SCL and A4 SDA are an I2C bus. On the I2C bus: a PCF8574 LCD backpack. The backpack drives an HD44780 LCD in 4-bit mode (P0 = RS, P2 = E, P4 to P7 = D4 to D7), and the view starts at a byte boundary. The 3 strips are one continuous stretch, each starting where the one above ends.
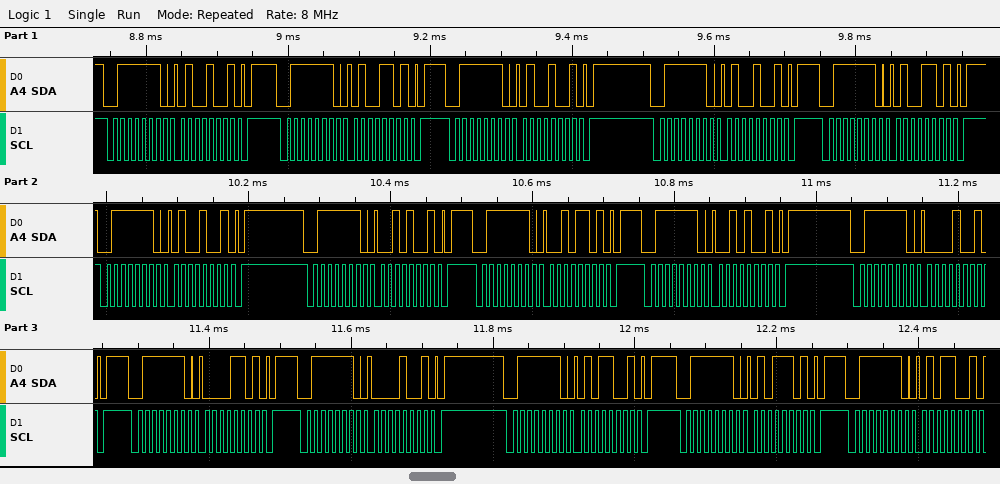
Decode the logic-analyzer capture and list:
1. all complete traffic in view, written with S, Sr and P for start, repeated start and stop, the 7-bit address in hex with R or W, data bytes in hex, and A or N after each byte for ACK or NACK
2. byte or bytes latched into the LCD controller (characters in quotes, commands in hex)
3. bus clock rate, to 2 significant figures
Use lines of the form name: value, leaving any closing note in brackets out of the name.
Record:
all complete traffic in view, written with S, Sr and P for start, repeated start and stop, the 7-bit address in hex with R or W, data bytes in hex, and A or N after each byte for ACK or NACK: S 3FW A 49 A P S 3FW A 4D A P S 3FW A 49 A P S 3FW A 49 A P S 3FW A 4D A P S 3FW A 49 A P S 3FW A 29 A P S 3FW A 2D A P S 3FW A 29 A P S 3FW A 09 A P S 3FW A 0D A P S 3FW A 09 A P S 3FW A 59 A P S 3FW A 5D A P S 3FW A 59 A
byte or bytes latched into the LCD controller: 'D' ' '
bus clock rate, to 2 significant figures: 100 kHz
